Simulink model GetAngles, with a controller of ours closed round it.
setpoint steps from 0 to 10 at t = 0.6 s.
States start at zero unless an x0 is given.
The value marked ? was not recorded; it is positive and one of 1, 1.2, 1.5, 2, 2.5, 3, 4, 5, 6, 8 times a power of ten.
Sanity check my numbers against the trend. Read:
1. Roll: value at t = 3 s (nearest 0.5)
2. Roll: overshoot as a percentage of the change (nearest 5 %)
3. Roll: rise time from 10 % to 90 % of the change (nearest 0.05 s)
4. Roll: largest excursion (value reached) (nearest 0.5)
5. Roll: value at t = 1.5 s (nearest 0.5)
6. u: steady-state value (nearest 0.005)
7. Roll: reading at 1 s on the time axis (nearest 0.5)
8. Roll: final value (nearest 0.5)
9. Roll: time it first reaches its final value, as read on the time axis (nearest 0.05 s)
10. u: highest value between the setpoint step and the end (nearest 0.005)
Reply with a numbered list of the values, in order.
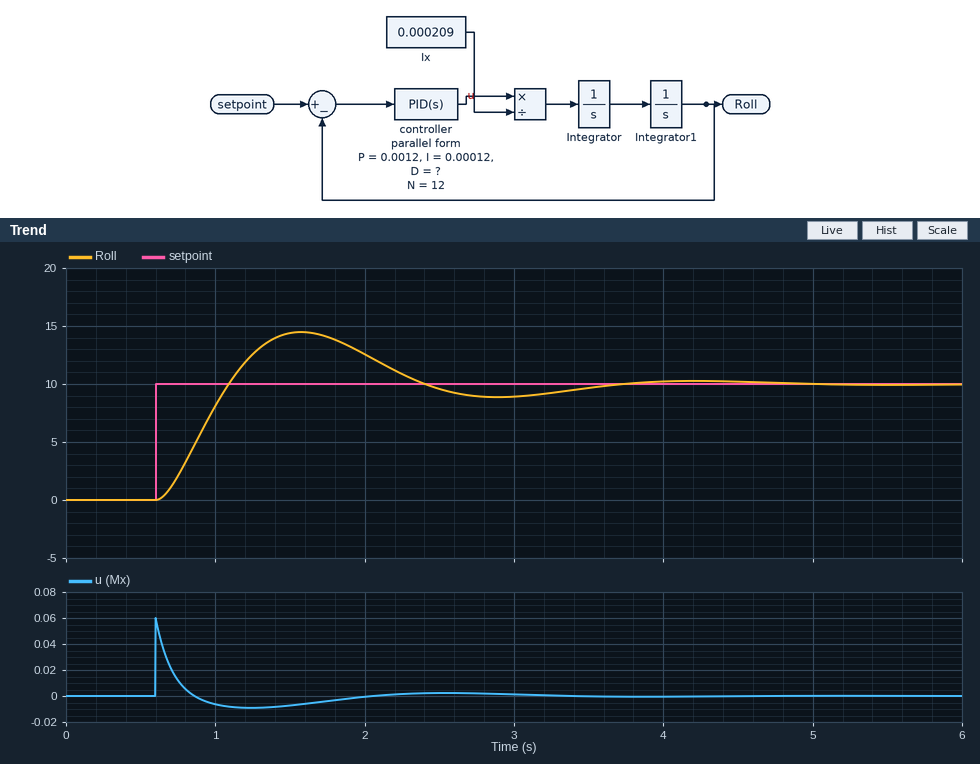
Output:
1. 9.0
2. 45 %
3. 0.35 s
4. 14.5
5. 14.5
6. 0.000
7. 8.0
8. 10.0
9. 1.10 s
10. 0.060
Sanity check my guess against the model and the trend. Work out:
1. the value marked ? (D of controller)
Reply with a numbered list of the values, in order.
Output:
1. 0.0004
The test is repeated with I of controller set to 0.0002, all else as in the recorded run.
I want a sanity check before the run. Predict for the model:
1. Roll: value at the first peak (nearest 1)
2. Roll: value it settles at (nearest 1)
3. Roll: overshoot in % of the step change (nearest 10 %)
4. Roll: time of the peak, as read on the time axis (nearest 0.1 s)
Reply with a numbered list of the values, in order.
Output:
1. 15
2. 10
3. 50 %
4. 1.6 s
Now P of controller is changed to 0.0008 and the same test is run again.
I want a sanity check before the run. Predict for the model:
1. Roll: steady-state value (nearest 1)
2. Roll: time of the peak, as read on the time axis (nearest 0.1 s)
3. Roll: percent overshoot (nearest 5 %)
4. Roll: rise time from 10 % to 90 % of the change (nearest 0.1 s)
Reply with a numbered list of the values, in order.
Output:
1. 10
2. 1.7 s
3. 40 %
4. 0.4 s
